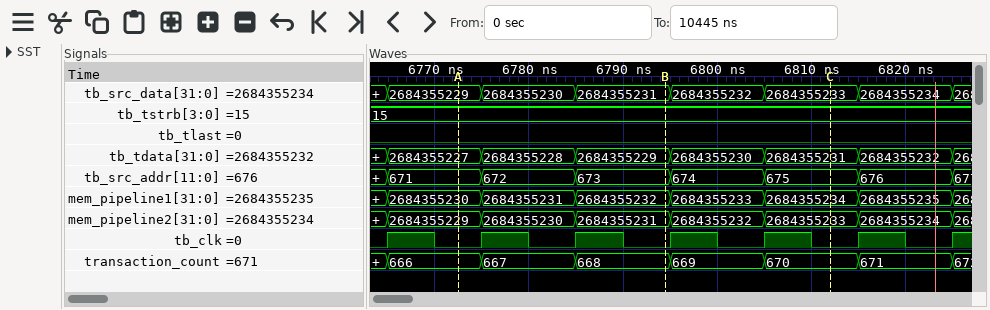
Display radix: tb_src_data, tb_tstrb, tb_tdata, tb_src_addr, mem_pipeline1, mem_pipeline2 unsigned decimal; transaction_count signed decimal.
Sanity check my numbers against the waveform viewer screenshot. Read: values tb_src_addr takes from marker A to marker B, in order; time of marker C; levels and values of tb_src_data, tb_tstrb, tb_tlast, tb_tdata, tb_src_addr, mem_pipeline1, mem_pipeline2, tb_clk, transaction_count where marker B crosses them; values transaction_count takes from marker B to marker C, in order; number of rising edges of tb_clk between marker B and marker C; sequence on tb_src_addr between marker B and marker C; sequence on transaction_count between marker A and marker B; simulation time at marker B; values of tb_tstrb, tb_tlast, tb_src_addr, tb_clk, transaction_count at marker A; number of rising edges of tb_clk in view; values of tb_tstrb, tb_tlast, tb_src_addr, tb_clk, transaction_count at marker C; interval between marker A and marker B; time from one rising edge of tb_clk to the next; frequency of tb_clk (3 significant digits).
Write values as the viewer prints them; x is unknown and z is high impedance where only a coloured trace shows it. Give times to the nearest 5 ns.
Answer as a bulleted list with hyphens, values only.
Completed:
- 671, 672, 673
- 6810 ns
- tb_src_data=2684355231, tb_tstrb=15, tb_tlast=0, tb_tdata=2684355229, tb_src_addr=673, mem_pipeline1=2684355232, mem_pipeline2=2684355231, tb_clk=0, transaction_count=668
- 668, 669, 670
- 2
- 673, 674, 675
- 666, 667, 668
- 6795 ns
- tb_tstrb=15, tb_tlast=0, tb_src_addr=671, tb_clk=0, transaction_count=666
- 7
- tb_tstrb=15, tb_tlast=0, tb_src_addr=675, tb_clk=0, transaction_count=670
- 20 ns
- 10 ns
- 100 MHz
